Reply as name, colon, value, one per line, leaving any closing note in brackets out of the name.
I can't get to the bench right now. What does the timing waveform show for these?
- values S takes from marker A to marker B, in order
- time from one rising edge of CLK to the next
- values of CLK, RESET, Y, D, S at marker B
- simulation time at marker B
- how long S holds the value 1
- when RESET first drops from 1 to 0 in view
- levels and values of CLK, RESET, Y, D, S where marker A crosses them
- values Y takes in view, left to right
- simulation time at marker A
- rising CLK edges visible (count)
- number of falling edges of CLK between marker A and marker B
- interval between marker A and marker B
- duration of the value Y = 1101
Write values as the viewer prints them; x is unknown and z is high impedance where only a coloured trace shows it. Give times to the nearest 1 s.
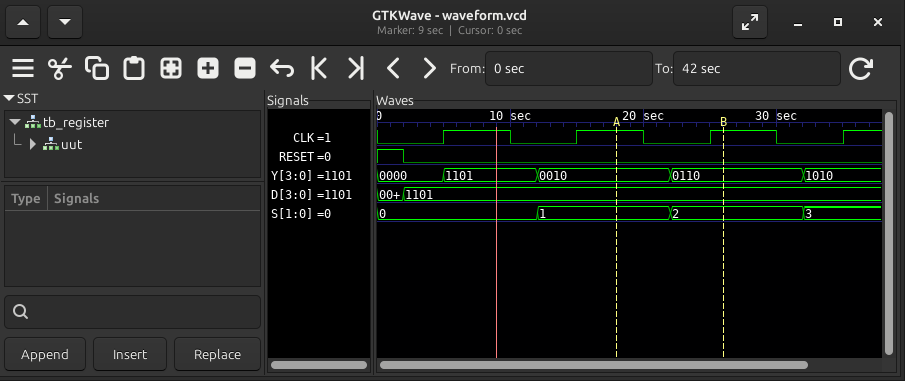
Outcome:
values S takes from marker A to marker B, in order: 1, 2
time from one rising edge of CLK to the next: 10 s
values of CLK, RESET, Y, D, S at marker B: CLK=1, RESET=0, Y=0110, D=1101, S=2
simulation time at marker B: 26 s
how long S holds the value 1: 10 s
when RESET first drops from 1 to 0 in view: 2 s
levels and values of CLK, RESET, Y, D, S where marker A crosses them: CLK=1, RESET=0, Y=0010, D=1101, S=1
values Y takes in view, left to right: 0000, 1101, 0010, 0110, 1010
simulation time at marker A: 18 s
rising CLK edges visible: 4
number of falling edges of CLK between marker A and marker B: 1
interval between marker A and marker B: 8 s
duration of the value Y = 1101: 7 s
